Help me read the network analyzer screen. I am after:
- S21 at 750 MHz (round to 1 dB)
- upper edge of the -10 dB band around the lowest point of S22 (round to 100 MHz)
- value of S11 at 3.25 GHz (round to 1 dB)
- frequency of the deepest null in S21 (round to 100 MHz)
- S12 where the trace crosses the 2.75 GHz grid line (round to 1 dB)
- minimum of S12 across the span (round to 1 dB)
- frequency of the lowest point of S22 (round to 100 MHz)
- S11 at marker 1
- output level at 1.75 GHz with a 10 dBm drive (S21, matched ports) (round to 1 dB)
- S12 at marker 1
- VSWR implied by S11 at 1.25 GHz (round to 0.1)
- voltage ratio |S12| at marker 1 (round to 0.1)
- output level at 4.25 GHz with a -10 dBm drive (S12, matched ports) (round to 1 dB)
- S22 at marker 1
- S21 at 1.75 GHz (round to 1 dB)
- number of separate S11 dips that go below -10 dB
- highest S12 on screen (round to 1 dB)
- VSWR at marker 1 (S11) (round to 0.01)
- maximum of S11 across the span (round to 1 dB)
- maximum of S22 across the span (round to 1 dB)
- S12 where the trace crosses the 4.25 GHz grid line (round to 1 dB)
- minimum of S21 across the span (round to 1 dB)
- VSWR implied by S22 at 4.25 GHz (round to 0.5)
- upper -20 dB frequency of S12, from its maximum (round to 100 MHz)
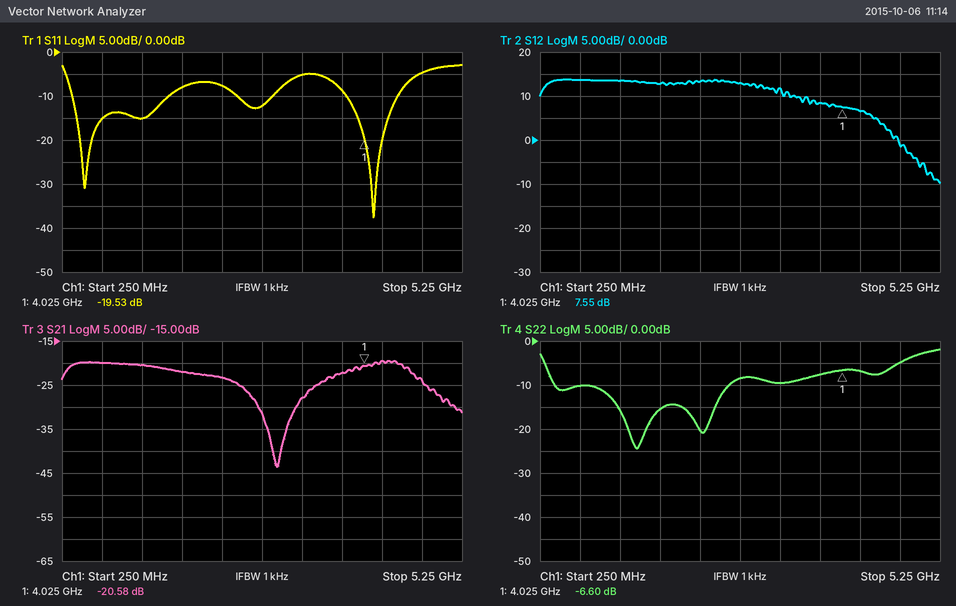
-20 dB
2.6 GHz
-5 dB
2.9 GHz
13 dB
-10 dB
1.5 GHz
-19.53 dB
-12 dBm
7.55 dB
1.4
2.4
-3 dBm
-6.60 dB
-22 dB
3
14 dB
1.24
-3 dB
-2 dB
7 dB
-44 dB
2.5
5.1 GHz
